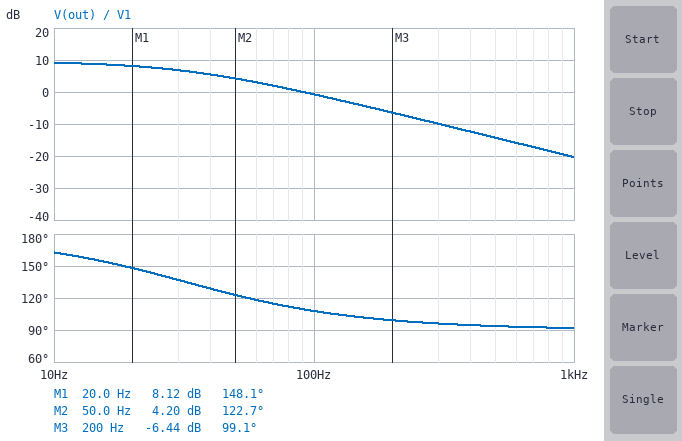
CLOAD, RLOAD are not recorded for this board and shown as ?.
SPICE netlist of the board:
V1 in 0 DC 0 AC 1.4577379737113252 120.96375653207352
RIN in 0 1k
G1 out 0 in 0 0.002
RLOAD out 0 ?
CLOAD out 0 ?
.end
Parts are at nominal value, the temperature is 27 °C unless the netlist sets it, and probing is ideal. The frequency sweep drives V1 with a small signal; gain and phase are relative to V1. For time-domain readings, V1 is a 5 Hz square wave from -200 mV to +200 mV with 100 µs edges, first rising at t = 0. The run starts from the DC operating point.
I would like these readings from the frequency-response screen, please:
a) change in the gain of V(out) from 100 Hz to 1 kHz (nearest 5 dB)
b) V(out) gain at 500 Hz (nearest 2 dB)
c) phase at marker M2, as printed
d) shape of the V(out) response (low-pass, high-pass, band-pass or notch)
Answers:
-20 dB
-14 dB
122.7 deg
low-pass
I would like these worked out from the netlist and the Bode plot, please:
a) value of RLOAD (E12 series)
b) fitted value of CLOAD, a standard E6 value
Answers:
1.5 kΩ
3.3 µF
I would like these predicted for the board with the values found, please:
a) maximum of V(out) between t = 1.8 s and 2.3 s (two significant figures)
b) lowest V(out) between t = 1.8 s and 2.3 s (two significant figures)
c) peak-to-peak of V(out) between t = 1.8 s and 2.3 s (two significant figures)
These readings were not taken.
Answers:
600 mV
-600 mV
1.2 V
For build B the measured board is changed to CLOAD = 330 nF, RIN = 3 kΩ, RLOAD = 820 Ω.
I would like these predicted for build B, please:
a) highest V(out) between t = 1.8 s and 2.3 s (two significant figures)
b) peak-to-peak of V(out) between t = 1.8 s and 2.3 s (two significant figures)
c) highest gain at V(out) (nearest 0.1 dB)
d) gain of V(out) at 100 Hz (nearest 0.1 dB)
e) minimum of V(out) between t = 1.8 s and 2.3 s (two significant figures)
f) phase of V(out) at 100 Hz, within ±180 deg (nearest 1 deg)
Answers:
330 mV
660 mV
4.3 dB
4.2 dB
-330 mV
170 deg
